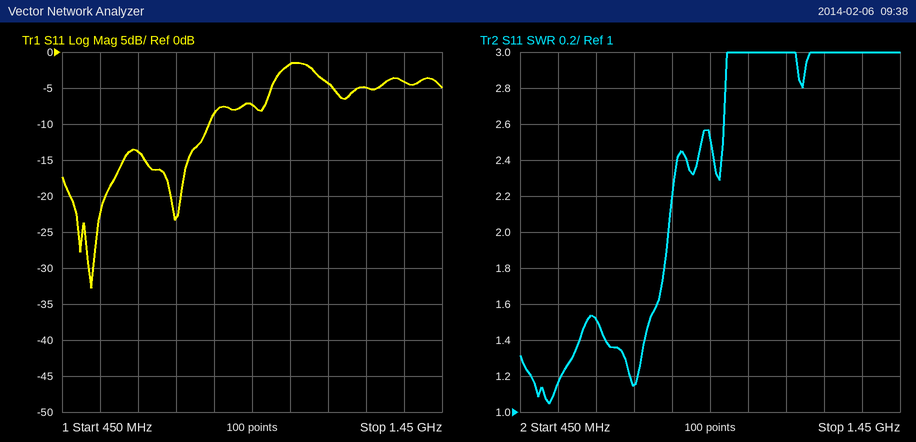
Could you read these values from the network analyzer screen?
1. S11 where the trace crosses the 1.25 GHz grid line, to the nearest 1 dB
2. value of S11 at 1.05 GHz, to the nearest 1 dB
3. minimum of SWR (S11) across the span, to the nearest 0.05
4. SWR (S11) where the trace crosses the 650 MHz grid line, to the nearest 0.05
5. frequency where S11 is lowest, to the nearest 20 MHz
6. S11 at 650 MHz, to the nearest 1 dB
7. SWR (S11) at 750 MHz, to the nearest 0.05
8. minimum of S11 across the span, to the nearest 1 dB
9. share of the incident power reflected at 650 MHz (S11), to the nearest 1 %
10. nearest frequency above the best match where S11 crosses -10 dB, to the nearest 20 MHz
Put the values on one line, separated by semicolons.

-5 dB; -2 dB; 1.05; 1.50; 520 MHz; -14 dB; 1.15; -33 dB; 4 %; 840 MHz
